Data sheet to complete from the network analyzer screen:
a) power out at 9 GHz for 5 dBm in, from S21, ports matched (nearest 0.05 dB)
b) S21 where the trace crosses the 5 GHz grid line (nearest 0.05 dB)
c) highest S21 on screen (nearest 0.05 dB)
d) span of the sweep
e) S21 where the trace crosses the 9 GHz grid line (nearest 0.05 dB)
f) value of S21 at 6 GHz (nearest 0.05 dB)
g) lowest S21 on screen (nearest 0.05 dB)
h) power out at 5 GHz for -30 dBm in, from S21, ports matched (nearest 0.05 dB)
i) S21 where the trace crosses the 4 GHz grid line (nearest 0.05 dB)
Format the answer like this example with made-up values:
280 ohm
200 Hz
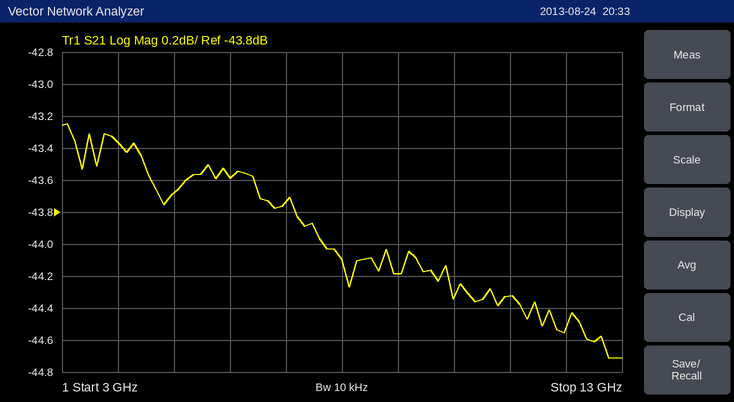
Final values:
-39.20 dBm
-43.70 dB
-43.25 dB
10 GHz
-44.20 dB
-43.60 dB
-44.70 dB
-73.70 dBm
-43.35 dB
